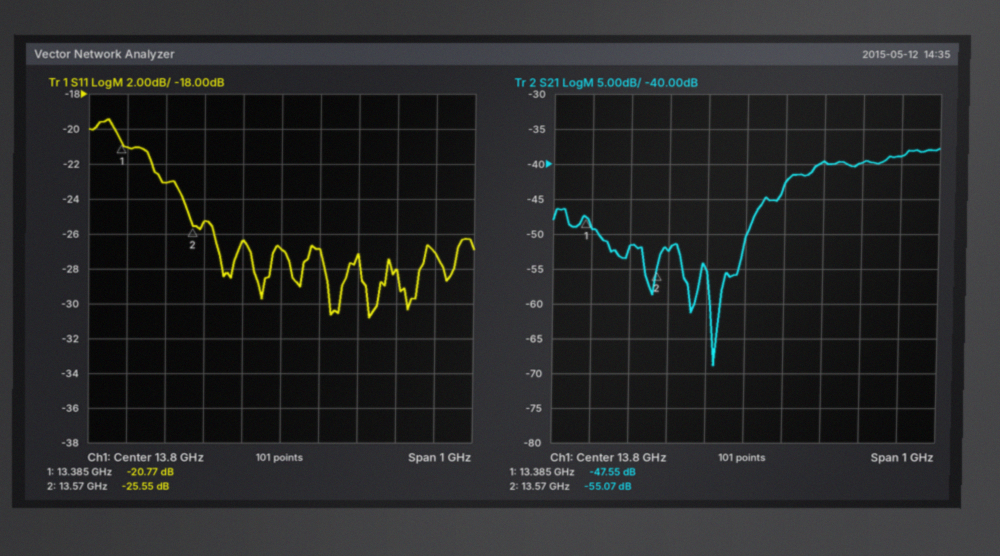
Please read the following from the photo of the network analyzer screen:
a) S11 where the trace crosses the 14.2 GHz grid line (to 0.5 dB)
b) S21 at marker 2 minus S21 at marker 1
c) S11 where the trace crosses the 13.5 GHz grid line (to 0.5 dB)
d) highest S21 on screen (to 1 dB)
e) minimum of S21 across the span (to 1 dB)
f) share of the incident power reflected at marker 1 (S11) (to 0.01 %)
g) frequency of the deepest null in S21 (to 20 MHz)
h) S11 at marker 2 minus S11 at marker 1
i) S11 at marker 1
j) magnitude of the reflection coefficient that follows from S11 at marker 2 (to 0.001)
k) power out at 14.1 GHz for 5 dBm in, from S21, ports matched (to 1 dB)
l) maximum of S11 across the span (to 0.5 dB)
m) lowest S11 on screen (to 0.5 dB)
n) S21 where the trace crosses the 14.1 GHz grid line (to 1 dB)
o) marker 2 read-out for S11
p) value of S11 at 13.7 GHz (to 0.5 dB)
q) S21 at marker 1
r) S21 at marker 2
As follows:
-27.0 dB
-7.52 dB
-23.0 dB
-38 dB
-69 dB
0.84 %
13.72 GHz
-4.78 dB
-20.77 dB
0.053
-35 dBm
-19.5 dB
-31.0 dB
-40 dB
-25.55 dB
-26.5 dB
-47.55 dB
-55.07 dB
